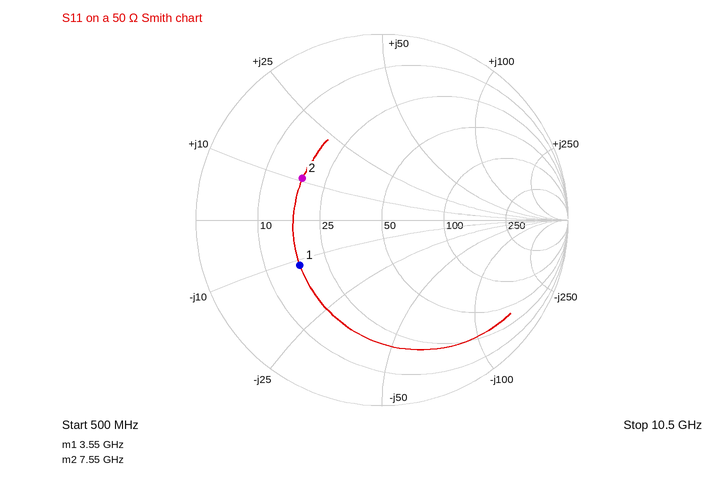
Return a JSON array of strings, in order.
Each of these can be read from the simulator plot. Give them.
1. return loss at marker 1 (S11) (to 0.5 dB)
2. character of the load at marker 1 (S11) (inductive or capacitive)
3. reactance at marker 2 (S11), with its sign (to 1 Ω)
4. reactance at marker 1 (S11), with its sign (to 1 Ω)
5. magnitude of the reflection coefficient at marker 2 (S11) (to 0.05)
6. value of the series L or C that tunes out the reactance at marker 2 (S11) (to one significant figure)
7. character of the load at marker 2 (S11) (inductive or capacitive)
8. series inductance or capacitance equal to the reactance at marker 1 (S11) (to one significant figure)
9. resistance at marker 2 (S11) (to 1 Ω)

["6.0 dB", "capacitive", "+11 Ω", "-11 Ω", "0.50", "2 pF", "inductive", "4 pF", "18 Ω"]
